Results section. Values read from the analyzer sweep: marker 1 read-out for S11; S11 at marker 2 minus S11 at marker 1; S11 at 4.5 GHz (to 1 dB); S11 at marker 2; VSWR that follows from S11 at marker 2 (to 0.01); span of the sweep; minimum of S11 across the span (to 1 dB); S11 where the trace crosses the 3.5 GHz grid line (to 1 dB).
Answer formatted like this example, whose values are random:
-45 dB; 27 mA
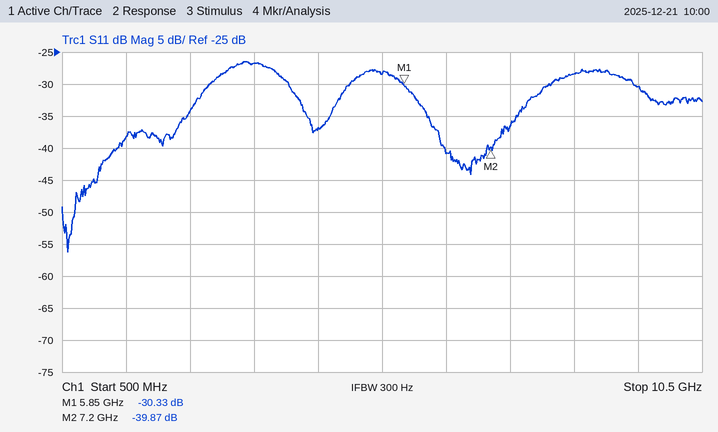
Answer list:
-30.33 dB; -9.54 dB; -37 dB; -39.87 dB; 1.02; 10 GHz; -56 dB; -27 dB
